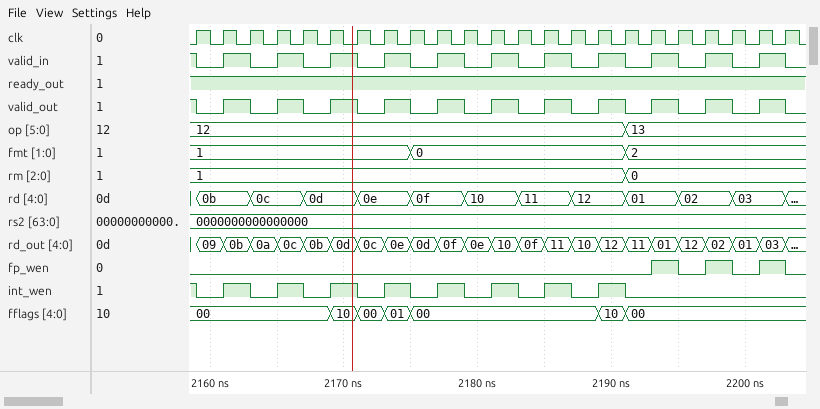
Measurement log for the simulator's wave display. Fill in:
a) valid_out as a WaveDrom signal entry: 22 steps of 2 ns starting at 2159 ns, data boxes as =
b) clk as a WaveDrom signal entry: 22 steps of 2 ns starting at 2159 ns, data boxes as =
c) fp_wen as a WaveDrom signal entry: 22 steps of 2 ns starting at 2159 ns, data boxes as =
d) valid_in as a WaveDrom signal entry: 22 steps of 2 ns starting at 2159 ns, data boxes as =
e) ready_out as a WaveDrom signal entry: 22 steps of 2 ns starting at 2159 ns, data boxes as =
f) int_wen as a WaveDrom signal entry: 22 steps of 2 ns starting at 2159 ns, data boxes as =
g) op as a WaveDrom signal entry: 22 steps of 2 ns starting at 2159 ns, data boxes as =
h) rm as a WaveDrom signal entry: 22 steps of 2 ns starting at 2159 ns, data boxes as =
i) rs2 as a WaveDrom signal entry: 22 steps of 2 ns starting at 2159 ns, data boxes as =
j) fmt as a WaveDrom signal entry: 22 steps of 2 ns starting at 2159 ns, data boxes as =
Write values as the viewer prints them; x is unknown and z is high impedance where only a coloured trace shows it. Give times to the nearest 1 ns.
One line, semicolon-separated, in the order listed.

{name: 'valid_out', wave: '0101010101010101010101'}; {name: 'clk', wave: 'p.....................'}; {name: 'fp_wen', wave: '0................10101'}; {name: 'valid_in', wave: '0101010101010101010101'}; {name: 'ready_out', wave: '1.....................'}; {name: 'int_wen', wave: '01010101010101010.....'}; {name: 'op', wave: '=...............=.....', data: '12 13'}; {name: 'rm', wave: '=...............=.....', data: '1 0'}; {name: 'rs2', wave: '=.....................', data: '0000000000000000'}; {name: 'fmt', wave: '=.......=.......=.....', data: '1 0 2'}
